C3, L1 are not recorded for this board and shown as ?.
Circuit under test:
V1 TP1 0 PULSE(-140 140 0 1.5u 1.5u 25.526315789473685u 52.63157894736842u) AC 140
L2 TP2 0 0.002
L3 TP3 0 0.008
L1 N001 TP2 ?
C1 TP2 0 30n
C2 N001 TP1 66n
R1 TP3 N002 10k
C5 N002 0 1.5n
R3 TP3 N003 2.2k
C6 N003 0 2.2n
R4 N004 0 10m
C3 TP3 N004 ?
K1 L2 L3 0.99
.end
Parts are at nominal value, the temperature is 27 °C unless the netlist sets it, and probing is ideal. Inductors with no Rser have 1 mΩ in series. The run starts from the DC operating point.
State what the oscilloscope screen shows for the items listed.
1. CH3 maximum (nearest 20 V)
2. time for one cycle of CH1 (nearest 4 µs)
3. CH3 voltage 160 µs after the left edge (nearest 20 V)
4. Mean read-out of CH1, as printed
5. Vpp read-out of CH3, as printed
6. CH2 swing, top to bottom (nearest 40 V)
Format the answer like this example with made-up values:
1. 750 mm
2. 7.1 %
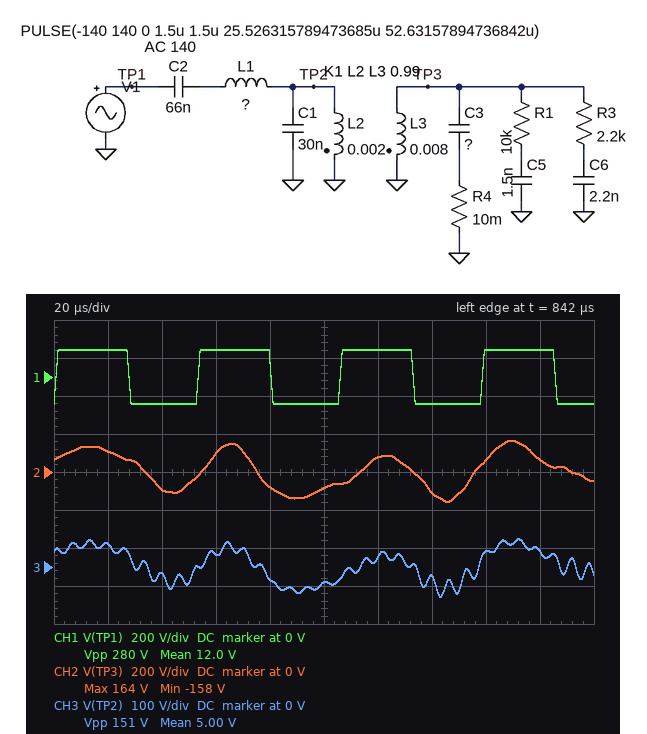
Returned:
1. 80 V
2. 52 µs
3. 40 V
4. 12.0 V
5. 151 V
6. 320 V
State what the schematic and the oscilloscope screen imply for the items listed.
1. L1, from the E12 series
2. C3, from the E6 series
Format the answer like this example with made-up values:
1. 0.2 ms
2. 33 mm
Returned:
1. 470 µH
2. 68 nF
